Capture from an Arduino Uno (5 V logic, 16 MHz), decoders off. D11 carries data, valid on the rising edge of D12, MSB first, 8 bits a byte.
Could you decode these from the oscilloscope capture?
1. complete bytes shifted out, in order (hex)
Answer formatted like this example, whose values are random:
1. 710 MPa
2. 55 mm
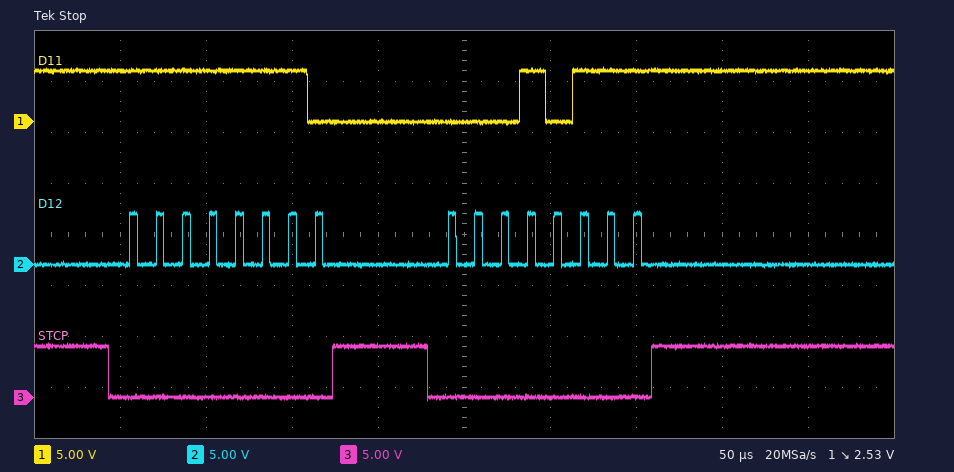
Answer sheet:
1. 0xFE 0x17
